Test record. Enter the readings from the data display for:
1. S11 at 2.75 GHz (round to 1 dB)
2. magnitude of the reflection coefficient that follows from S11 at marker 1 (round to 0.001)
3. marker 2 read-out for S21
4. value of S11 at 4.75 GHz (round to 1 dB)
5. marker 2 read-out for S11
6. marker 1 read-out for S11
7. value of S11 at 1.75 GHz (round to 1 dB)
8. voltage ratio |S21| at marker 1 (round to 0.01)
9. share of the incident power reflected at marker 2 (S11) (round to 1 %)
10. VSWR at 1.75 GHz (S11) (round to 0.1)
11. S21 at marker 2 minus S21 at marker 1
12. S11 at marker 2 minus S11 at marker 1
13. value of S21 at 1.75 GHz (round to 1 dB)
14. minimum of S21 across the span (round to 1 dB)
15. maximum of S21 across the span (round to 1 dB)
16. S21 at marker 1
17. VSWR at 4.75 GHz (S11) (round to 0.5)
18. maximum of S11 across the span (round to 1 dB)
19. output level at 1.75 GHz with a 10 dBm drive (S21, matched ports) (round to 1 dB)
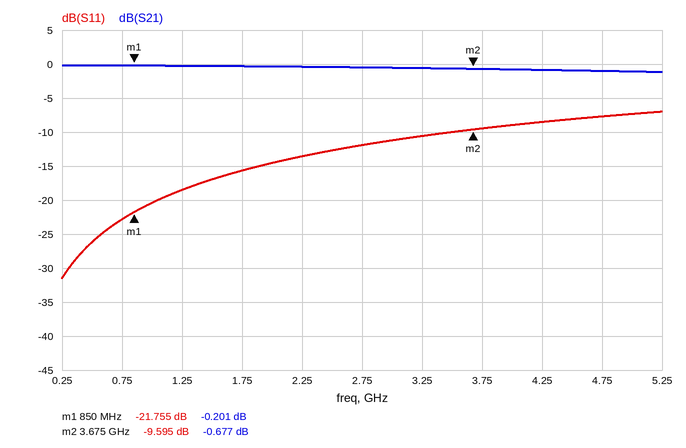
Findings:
-12 dB
0.082
-0.677 dB
-8 dB
-9.595 dB
-21.755 dB
-16 dB
0.98
11 %
1.4
-0.476 dB
12.160 dB
0 dB
-1 dB
0 dB
-0.201 dB
2.5
-7 dB
10 dBm
